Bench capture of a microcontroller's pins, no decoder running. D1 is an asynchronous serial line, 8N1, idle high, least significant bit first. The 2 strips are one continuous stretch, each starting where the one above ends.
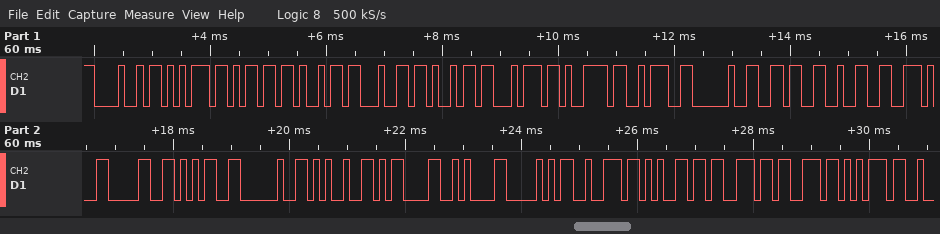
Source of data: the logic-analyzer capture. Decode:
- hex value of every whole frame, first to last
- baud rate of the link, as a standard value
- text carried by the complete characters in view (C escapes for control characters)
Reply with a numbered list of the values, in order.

1. 0x48 0x75 0x6D 0x69 0x64 0x69 0x74 0x79 0x3A 0x20 0x36 0x32 0x2E 0x30 0x35 0x20 0x25 0x0D 0x0A 0x50 0x72 0x65 0x73 0x73 0x75
2. 9600 baud
3. "Humidity: 62.05 %\r\nPressu"
